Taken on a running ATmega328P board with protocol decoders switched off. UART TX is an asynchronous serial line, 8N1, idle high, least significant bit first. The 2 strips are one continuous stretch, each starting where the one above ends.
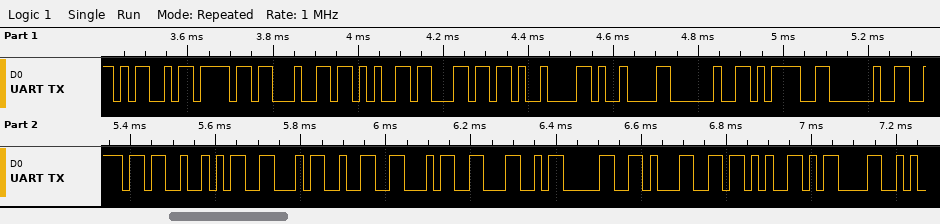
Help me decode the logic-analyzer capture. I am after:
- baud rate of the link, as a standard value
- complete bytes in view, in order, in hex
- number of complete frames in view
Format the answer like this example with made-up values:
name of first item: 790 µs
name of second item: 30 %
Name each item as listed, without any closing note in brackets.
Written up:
baud rate of the link, as a standard value: 57600 baud
complete bytes in view, in order, in hex: 4D 6F 64 65 6C 09 09 20 3D 20 6E 52 46 32 34 4C 30 31 2B 0D
number of complete frames in view: 20
